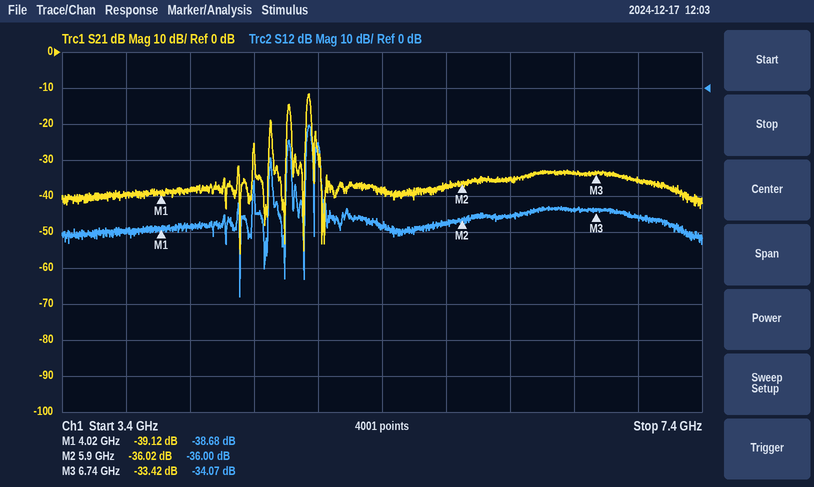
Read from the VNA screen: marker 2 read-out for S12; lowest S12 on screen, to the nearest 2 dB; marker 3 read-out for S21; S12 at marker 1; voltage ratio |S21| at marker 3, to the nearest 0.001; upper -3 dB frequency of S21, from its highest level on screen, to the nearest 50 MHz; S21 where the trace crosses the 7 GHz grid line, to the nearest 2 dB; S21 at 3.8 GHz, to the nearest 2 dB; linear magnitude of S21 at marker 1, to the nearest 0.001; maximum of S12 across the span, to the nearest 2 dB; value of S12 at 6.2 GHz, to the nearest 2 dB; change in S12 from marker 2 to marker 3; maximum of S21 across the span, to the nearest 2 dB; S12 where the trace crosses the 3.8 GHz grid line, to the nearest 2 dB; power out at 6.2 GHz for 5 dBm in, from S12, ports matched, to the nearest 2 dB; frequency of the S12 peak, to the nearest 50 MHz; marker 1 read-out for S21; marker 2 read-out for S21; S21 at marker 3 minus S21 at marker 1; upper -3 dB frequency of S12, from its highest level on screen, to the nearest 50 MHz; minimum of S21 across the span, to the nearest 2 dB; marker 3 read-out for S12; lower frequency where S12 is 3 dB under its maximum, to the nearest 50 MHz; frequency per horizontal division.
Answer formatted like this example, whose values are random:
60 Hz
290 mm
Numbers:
-36.00 dB
-58 dB
-33.42 dB
-38.68 dB
0.021
4.95 GHz
-36 dB
-40 dB
0.011
-10 dB
-36 dB
1.93 dB
-12 dB
-40 dB
-30 dBm
4.95 GHz
-39.12 dB
-36.02 dB
5.70 dB
4.95 GHz
-56 dB
-34.07 dB
4.95 GHz
400 MHz
